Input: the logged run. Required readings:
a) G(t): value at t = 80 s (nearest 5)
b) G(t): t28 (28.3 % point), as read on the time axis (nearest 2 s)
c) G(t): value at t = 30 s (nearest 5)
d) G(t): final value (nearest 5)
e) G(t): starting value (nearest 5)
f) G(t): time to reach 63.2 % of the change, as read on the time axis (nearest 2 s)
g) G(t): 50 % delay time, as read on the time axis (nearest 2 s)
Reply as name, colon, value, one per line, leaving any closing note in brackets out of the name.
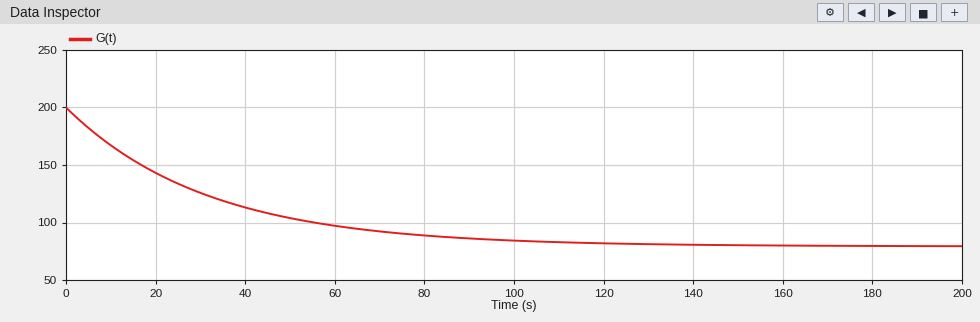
G(t): value at t = 80 s: 90
G(t): t28 (28.3 % point), as read on the time axis: 10 s
G(t): value at t = 30 s: 125
G(t): final value: 80
G(t): starting value: 200
G(t): time to reach 63.2 % of the change, as read on the time axis: 32 s
G(t): 50 % delay time, as read on the time axis: 22 s
